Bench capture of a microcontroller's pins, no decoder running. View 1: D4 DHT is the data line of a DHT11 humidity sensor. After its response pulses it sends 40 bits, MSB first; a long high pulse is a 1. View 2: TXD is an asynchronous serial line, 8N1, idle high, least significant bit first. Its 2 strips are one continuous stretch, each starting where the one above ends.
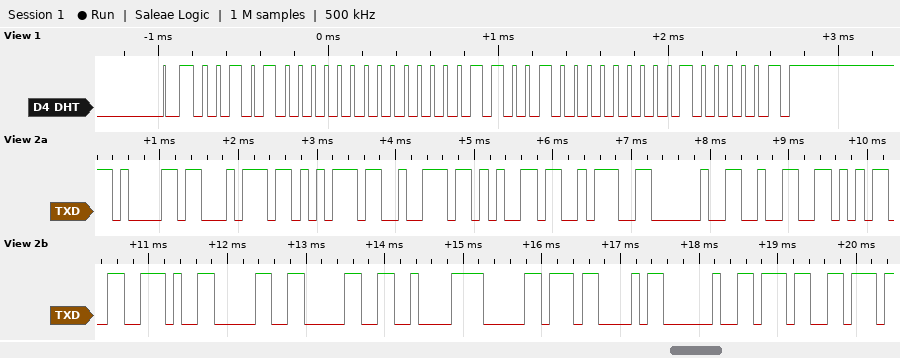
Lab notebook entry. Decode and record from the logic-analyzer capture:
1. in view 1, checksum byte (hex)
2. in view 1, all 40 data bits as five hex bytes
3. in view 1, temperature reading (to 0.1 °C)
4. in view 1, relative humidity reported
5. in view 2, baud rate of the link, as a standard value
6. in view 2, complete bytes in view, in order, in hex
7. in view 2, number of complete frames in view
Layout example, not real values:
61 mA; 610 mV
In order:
0x41; 28 00 19 00 41; 25.0 °C; 40 %; 9600 baud; 61 74 75 72 65 3A 20 32 35 2E 30 30 C2 B0 43 20 37; 17
